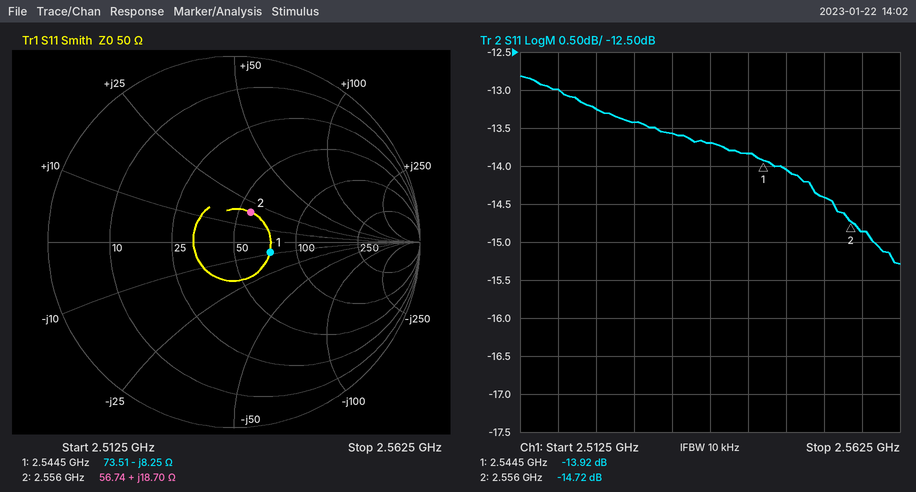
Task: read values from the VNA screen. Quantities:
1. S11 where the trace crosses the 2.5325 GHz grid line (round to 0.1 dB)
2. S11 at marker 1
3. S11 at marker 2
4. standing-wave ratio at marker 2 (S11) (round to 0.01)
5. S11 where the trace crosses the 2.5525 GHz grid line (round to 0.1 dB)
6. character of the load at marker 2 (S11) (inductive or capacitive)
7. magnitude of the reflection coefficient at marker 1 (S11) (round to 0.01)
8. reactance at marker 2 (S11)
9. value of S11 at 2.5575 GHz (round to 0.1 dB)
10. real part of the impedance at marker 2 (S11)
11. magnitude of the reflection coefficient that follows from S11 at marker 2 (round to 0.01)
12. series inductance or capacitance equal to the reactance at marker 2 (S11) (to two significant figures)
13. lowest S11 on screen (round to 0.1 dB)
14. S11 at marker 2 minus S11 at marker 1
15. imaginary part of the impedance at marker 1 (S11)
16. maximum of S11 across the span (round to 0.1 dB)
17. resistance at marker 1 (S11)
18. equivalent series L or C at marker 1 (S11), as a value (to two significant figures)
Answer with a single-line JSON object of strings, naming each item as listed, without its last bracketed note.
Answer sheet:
{"S11 where the trace crosses the 2.5325 GHz grid line": "-13.6 dB", "S11 at marker 1": "-13.92 dB", "S11 at marker 2": "-14.72 dB", "standing-wave ratio at marker 2 (S11)": "1.45", "S11 where the trace crosses the 2.5525 GHz grid line": "-14.4 dB", "character of the load at marker 2 (S11)": "inductive", "magnitude of the reflection coefficient at marker 1 (S11)": "0.20", "reactance at marker 2": "+18.70 Ω", "value of S11 at 2.5575 GHz": "-14.9 dB", "real part of the impedance at marker 2": "56.74 Ω", "magnitude of the reflection coefficient that follows from S11 at marker 2": "0.18", "series inductance or capacitance equal to the reactance at marker 2 (S11)": "1.2 nH", "lowest S11 on screen": "-15.3 dB", "S11 at marker 2 minus S11 at marker 1": "-0.80 dB", "imaginary part of the impedance at marker 1": "-8.25 Ω", "maximum of S11 across the span": "-12.8 dB", "resistance at marker 1": "73.51 Ω", "equivalent series L or C at marker 1 (S11), as a value": "7.6 pF"}
